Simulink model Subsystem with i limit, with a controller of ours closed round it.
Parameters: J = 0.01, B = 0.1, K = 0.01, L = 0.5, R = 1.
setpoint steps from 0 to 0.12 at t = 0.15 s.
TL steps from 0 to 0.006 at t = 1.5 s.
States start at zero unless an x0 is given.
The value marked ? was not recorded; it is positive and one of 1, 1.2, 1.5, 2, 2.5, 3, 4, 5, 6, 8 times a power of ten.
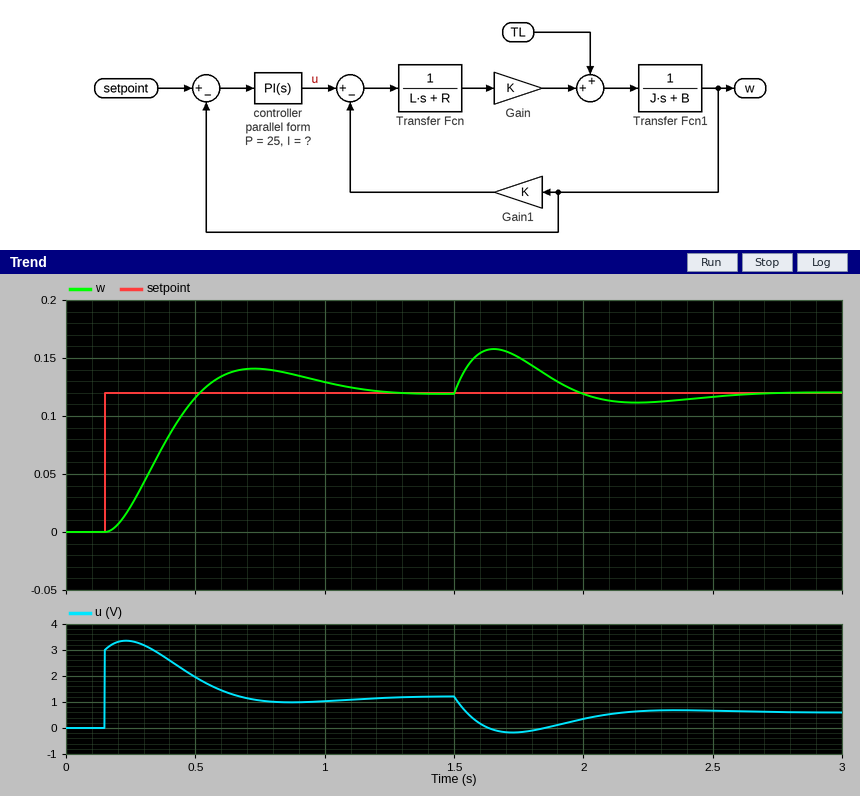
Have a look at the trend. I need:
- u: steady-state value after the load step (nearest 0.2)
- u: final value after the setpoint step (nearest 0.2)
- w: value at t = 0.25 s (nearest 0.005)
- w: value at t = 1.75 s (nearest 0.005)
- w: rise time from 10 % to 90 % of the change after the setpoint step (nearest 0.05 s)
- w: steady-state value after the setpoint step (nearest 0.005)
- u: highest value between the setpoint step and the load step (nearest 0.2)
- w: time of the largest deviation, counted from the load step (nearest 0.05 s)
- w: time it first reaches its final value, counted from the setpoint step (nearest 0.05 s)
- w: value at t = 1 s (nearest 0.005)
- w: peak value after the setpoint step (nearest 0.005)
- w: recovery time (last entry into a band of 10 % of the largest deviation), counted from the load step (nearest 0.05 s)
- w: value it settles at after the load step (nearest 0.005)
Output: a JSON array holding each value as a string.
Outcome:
["0.6", "1.2", "0.020", "0.150", "0.25 s", "0.120", "3.4", "0.15 s", "0.35 s", "0.130", "0.140", "1.00 s", "0.120"]
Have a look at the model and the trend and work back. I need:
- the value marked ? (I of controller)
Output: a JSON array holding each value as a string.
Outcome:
["80"]
